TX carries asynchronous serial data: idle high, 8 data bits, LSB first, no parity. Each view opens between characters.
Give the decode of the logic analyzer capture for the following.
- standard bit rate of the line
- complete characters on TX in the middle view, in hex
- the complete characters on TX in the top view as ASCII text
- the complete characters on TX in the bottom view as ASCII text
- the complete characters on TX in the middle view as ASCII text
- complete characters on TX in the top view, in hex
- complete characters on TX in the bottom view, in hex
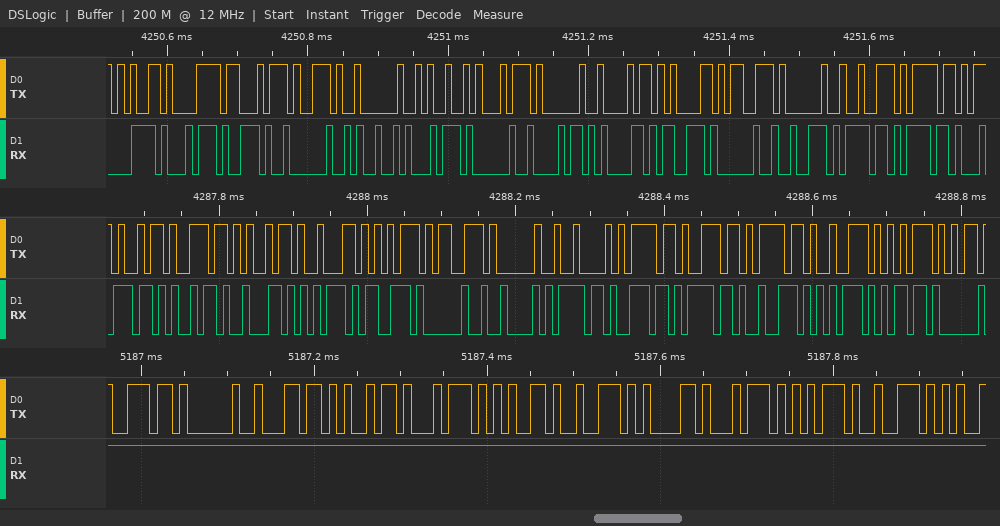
115200 baud
69, 6E, 69, 62, 75, 73, 20, 42, 6F, 6E, 6F, 72, 75
"ext. It has ro"
"n literatur"
"inibus Bonoru"
65, 78, 74, 2E, 20, 49, 74, 20, 68, 61, 73, 20, 72, 6F
6E, 20, 6C, 69, 74, 65, 72, 61, 74, 75, 72
